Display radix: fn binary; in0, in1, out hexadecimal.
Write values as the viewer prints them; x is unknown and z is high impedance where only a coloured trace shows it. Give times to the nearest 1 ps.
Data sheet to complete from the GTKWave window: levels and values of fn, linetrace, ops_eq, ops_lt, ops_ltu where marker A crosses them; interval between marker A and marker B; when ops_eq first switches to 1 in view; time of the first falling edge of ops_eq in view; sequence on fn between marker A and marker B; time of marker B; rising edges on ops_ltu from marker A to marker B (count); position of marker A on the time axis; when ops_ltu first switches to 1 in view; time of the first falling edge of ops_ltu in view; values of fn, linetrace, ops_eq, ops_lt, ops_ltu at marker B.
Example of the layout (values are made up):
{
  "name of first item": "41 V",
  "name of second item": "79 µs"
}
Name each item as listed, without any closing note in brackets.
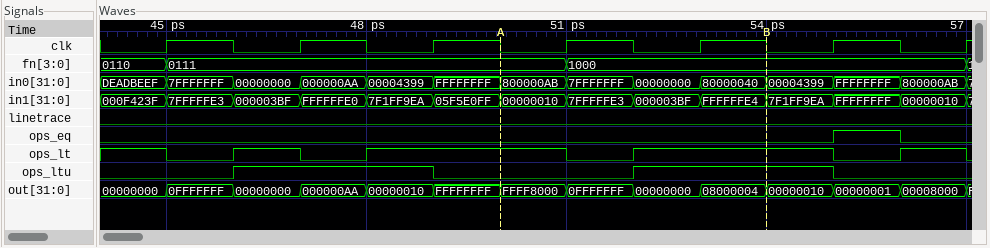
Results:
{
  "levels and values of fn, linetrace, ops_eq, ops_lt, ops_ltu where marker A crosses them": "fn=0111, linetrace=0, ops_eq=0, ops_lt=1, ops_ltu=0",
  "interval between marker A and marker B": "4 ps",
  "when ops_eq first switches to 1 in view": "55 ps",
  "time of the first falling edge of ops_eq in view": "56 ps",
  "sequence on fn between marker A and marker B": "0111, 1000",
  "time of marker B": "54 ps",
  "rising edges on ops_ltu from marker A to marker B": "1",
  "position of marker A on the time axis": "50 ps",
  "when ops_ltu first switches to 1 in view": "46 ps",
  "time of the first falling edge of ops_ltu in view": "49 ps",
  "values of fn, linetrace, ops_eq, ops_lt, ops_ltu at marker B": "fn=1000, linetrace=0, ops_eq=0, ops_lt=1, ops_ltu=1"
}
